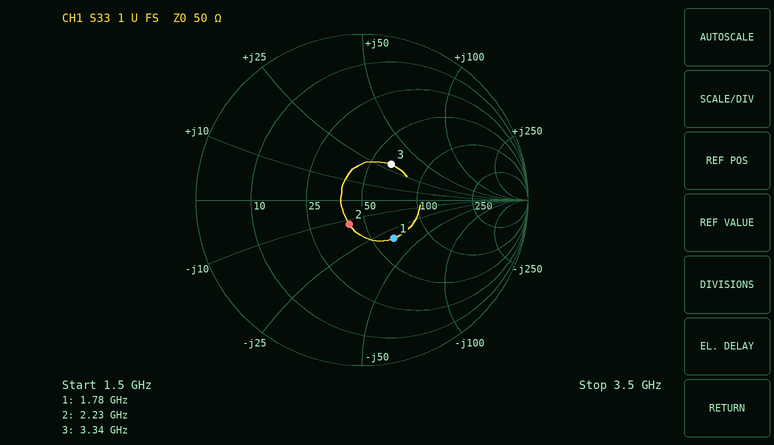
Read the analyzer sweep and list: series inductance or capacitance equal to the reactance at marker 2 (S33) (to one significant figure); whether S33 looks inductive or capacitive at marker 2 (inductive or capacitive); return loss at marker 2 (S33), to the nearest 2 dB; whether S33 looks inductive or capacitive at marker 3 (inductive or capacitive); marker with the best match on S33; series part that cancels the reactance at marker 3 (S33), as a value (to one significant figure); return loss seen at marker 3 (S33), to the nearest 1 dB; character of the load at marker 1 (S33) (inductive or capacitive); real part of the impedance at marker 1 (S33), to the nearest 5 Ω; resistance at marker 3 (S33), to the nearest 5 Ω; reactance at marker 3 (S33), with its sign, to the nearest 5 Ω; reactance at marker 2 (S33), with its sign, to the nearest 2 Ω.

6 pF
capacitive
16 dB
inductive
marker 2
2 pF
11 dB
capacitive
65 Ω
65 Ω
+30 Ω
-12 Ω
